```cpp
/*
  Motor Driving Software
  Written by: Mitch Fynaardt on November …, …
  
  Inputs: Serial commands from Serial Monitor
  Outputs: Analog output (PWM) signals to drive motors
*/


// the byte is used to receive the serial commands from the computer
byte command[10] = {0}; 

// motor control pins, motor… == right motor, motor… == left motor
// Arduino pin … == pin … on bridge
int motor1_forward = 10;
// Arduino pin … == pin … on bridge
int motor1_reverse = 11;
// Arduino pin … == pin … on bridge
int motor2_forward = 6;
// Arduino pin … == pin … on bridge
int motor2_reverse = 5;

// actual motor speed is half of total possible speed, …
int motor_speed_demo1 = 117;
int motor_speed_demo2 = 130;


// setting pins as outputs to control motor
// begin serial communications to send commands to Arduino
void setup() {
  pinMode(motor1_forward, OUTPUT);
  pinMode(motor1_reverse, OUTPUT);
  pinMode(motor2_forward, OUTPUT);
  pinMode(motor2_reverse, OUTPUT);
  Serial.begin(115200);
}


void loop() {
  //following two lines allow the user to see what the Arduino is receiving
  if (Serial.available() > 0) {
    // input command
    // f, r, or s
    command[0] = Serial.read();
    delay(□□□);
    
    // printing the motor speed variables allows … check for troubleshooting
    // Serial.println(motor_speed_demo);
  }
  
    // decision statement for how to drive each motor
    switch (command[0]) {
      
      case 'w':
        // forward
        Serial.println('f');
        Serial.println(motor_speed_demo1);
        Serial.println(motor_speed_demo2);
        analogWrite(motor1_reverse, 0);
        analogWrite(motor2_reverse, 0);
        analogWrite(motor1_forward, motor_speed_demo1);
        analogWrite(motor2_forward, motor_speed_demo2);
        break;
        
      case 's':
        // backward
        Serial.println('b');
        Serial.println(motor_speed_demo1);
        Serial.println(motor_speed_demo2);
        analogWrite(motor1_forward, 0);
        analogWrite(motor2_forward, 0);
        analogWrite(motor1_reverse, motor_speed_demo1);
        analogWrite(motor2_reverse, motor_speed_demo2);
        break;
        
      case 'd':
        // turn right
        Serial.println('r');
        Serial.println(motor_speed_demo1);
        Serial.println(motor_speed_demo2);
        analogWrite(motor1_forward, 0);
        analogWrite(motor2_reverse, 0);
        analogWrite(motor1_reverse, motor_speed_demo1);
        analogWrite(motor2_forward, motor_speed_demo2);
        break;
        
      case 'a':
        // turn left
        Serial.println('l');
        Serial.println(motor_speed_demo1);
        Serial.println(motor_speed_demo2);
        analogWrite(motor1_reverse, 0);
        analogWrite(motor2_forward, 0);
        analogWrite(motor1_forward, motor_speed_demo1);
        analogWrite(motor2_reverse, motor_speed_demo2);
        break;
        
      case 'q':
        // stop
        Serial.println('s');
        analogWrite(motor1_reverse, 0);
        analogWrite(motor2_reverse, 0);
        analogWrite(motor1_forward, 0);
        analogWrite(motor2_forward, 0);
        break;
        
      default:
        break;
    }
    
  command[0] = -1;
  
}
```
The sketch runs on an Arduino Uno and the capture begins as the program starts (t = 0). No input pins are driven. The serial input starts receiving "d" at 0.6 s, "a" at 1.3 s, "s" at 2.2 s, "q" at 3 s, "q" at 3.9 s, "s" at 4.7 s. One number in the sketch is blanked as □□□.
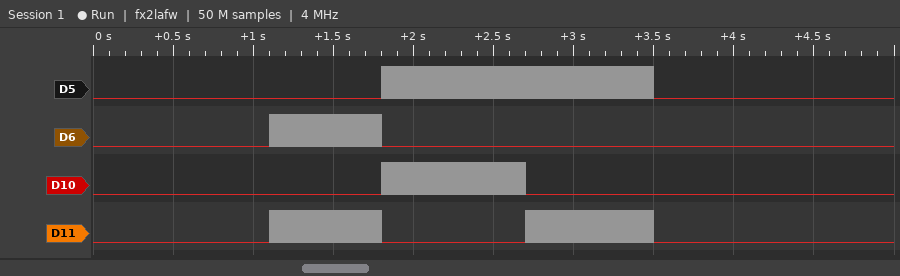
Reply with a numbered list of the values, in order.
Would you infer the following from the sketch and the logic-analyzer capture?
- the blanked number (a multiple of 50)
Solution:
1. 500
